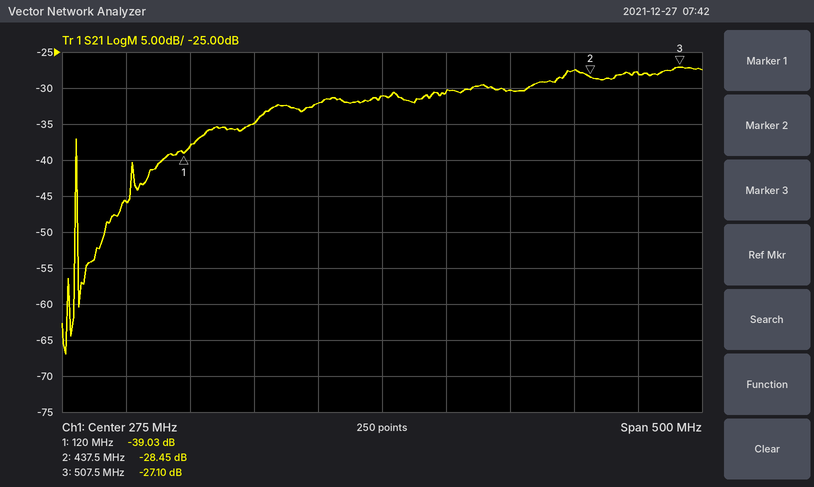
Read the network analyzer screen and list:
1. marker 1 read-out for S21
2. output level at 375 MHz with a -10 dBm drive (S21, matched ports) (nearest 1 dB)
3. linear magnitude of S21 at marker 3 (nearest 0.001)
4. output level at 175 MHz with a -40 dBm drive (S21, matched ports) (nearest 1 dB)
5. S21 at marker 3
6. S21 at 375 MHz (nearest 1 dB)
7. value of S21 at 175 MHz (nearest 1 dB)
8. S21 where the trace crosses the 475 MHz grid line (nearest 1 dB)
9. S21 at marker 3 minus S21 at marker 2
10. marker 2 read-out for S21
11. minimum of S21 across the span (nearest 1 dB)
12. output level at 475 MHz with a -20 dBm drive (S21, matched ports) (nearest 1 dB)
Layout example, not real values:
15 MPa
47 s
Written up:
-39.03 dB
-40 dBm
0.044
-75 dBm
-27.10 dB
-30 dB
-35 dB
-28 dB
1.35 dB
-28.45 dB
-67 dB
-48 dBm
